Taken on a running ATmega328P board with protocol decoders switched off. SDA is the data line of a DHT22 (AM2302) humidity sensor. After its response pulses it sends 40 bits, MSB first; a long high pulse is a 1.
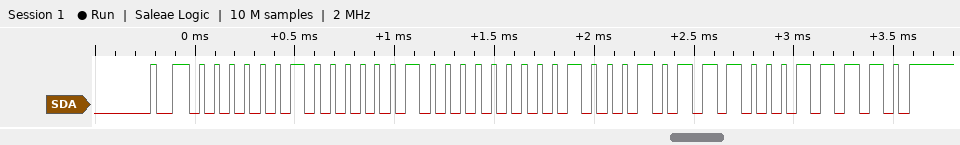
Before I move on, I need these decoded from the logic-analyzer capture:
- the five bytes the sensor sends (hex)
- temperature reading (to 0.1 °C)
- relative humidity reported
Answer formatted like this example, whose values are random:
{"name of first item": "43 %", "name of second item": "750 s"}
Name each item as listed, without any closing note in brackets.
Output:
{"the five bytes the sensor sends": "02 04 01 17 1E", "temperature reading": "27.9 °C", "relative humidity reported": "51.6 %"}
